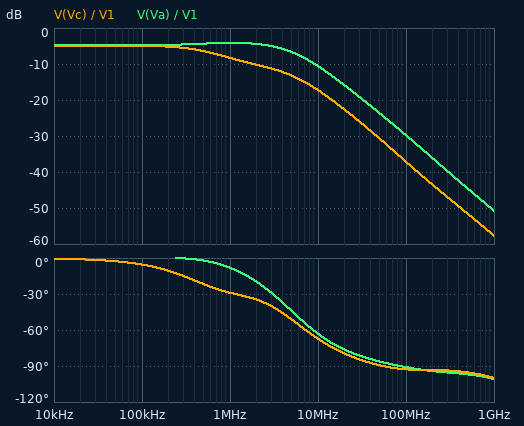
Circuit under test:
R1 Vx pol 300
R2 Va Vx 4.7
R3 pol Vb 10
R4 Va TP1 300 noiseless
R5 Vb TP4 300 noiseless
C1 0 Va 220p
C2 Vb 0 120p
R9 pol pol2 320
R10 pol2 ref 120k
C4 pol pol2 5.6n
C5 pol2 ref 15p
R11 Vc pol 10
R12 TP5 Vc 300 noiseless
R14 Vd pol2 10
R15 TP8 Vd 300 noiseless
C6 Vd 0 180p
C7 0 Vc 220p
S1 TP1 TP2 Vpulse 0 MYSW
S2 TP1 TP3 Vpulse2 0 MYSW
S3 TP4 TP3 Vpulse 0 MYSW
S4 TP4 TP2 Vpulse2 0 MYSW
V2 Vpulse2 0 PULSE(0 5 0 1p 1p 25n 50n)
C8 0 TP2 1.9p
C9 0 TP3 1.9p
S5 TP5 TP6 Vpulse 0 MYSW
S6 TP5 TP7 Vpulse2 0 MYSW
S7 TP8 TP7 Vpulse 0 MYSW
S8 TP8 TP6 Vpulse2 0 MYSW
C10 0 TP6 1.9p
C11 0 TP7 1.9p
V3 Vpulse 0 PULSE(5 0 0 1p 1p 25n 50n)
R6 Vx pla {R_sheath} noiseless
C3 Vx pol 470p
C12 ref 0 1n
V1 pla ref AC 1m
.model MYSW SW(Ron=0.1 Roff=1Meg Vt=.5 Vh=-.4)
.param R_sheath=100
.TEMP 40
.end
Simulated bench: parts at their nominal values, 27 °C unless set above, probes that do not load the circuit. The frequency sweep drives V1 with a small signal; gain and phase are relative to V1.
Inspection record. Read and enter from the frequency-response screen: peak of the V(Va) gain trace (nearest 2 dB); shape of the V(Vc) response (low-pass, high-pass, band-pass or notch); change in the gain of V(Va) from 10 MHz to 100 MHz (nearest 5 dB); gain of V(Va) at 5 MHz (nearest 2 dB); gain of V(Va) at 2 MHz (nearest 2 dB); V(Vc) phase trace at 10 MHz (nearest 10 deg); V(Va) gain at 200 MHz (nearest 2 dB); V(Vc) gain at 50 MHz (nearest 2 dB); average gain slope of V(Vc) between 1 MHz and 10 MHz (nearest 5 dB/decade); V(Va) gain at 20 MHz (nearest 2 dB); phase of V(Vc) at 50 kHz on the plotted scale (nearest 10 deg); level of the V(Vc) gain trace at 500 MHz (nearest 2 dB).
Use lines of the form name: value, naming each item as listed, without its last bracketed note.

peak of the V(Va) gain trace: -4 dB
shape of the V(Vc) response: low-pass
change in the gain of V(Va) from 10 MHz to 100 MHz: -20 dB
gain of V(Va) at 5 MHz: -6 dB
gain of V(Va) at 2 MHz: -4 dB
V(Vc) phase trace at 10 MHz: -70 deg
V(Va) gain at 200 MHz: -36 dB
V(Vc) gain at 50 MHz: -30 dB
average gain slope of V(Vc) between 1 MHz and 10 MHz: -10 dB/decade
V(Va) gain at 20 MHz: -16 dB
phase of V(Vc) at 50 kHz on the plotted scale: 0 deg
level of the V(Vc) gain trace at 500 MHz: -52 dB
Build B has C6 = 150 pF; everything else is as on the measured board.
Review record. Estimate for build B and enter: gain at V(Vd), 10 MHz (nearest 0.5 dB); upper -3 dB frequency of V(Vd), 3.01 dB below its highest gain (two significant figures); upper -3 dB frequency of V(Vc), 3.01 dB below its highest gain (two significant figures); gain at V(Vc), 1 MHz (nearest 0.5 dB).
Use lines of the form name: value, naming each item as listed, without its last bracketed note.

gain at V(Vd), 10 MHz: -17.0 dB
upper -3 dB frequency of V(Vd), 3.01 dB below its highest gain: 830 kHz
upper -3 dB frequency of V(Vc), 3.01 dB below its highest gain: 900 kHz
gain at V(Vc), 1 MHz: -8.0 dB
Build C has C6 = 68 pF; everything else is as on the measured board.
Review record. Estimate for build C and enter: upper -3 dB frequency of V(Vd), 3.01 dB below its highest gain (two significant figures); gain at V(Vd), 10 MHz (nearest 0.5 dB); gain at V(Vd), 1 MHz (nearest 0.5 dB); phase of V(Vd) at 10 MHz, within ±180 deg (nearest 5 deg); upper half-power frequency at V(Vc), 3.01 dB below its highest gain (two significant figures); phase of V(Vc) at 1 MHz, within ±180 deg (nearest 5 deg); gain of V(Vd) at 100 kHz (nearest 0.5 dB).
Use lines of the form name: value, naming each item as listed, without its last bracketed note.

upper -3 dB frequency of V(Vd), 3.01 dB below its highest gain: 980 kHz
gain at V(Vd), 10 MHz: -16.0 dB
gain at V(Vd), 1 MHz: -7.5 dB
phase of V(Vd) at 10 MHz, within ±180 deg: -60 deg
upper half-power frequency at V(Vc), 3.01 dB below its highest gain: 1.0 MHz
phase of V(Vc) at 1 MHz, within ±180 deg: -25 deg
gain of V(Vd) at 100 kHz: -4.5 dB
